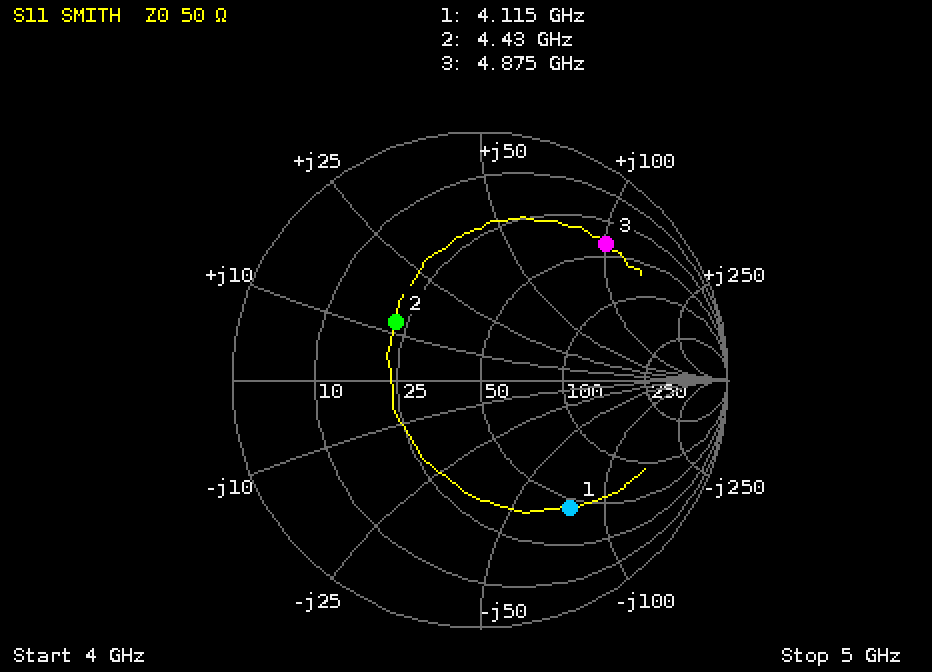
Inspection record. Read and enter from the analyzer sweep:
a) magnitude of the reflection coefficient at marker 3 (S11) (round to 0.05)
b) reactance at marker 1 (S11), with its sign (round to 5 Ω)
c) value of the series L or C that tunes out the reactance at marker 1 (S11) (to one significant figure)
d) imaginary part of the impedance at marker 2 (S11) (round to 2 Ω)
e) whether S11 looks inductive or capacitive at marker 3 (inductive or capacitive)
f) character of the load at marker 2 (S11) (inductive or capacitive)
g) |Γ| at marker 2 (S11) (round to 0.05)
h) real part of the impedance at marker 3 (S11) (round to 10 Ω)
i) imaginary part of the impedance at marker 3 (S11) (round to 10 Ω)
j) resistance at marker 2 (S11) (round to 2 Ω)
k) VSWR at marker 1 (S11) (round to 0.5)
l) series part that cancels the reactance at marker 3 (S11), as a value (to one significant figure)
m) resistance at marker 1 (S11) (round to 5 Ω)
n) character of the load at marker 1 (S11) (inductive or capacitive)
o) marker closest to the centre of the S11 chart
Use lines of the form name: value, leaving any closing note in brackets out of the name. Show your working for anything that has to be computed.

magnitude of the reflection coefficient at marker 3 (S11): 0.75
reactance at marker 1 (S11), with its sign: -75 Ω
value of the series L or C that tunes out the reactance at marker 1 (S11): L = 75 Ω/(2π × 4.115 GHz) ≈ 3 nH
imaginary part of the impedance at marker 2 (S11): +12 Ω
whether S11 looks inductive or capacitive at marker 3: inductive
character of the load at marker 2 (S11): inductive
|Γ| at marker 2 (S11): 0.40
real part of the impedance at marker 3 (S11): 40 Ω
imaginary part of the impedance at marker 3 (S11): +100 Ω
resistance at marker 2 (S11): 22 Ω
VSWR at marker 1 (S11): 4.5
series part that cancels the reactance at marker 3 (S11), as a value: C = 1/(2π × 4.875 GHz × 100 Ω) ≈ 326 fF, so 300 fF to one significant figure
resistance at marker 1 (S11): 45 Ω
character of the load at marker 1 (S11): capacitive
marker closest to the centre of the S11 chart: marker 2
